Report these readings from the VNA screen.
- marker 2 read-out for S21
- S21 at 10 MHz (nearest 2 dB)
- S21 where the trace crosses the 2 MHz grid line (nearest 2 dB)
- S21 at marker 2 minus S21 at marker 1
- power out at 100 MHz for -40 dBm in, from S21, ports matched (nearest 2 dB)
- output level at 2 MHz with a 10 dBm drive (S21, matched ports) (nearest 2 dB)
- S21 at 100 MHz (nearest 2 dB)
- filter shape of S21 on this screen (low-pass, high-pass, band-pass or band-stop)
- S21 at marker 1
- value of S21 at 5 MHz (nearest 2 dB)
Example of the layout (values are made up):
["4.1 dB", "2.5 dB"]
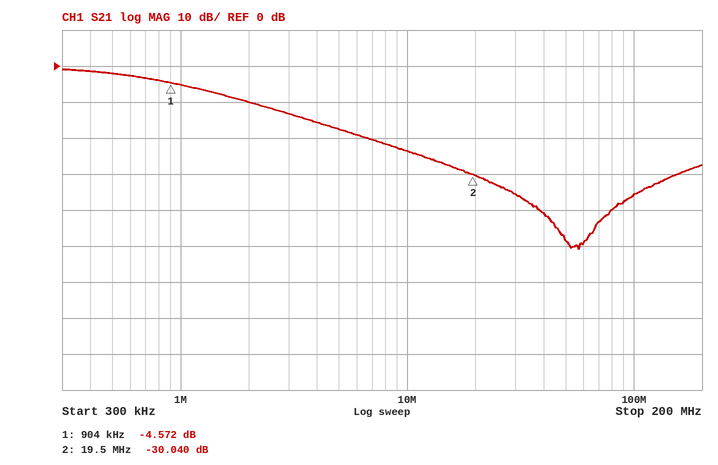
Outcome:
["-30.040 dB", "-24 dB", "-10 dB", "-25.468 dB", "-76 dBm", "0 dBm", "-36 dB", "low-pass", "-4.572 dB", "-18 dB"]
